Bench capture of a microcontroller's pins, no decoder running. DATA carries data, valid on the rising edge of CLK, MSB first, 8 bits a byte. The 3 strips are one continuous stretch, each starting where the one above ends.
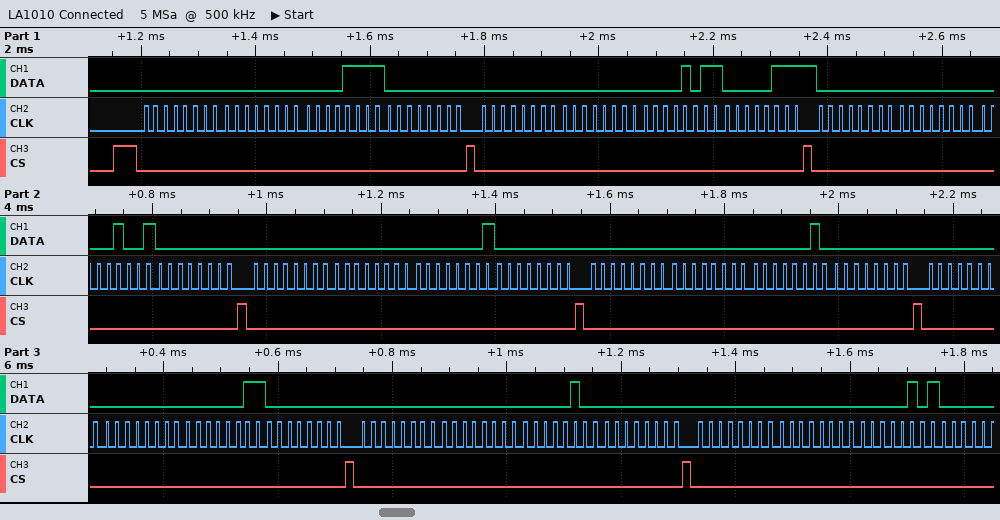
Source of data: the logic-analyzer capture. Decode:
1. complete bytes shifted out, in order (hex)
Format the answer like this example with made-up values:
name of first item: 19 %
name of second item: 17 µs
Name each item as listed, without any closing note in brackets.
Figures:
complete bytes shifted out, in order: 0x00 0x00 0x0F 0x00 0x00 0x00 0x0B 0x07 0x00 0x00 0x09 0x00 0x00 0x00 0x01 0x00 0x00 0x00 0x02 0x00 0x00 0x00 0x03 0x00 0x00 0x00 0x04 0x00 0x00 0x00 0x05
